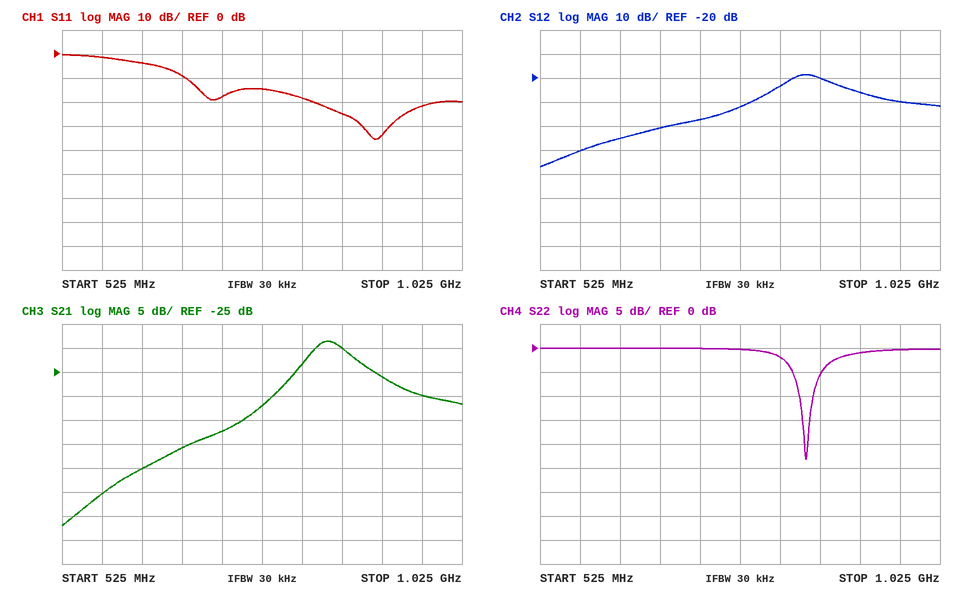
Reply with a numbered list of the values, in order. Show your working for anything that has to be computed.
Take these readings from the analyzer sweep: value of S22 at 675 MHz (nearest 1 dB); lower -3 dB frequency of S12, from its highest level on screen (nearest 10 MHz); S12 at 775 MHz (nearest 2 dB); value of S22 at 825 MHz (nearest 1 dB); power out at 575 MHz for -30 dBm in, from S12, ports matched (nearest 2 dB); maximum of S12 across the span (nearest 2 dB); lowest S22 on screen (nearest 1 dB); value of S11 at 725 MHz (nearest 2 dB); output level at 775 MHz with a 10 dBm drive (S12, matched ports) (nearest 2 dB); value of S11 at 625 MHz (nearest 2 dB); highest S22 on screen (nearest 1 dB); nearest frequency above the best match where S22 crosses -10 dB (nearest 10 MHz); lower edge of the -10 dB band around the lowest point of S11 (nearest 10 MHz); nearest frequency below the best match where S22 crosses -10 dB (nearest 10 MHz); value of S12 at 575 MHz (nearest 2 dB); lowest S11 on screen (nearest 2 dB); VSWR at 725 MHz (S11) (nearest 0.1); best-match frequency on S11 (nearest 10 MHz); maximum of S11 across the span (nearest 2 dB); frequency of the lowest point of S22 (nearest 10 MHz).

1. 0 dB
2. 830 MHz
3. -32 dB
4. -2 dB
5. -30 dBm + (-50 dB) = -80 dBm
6. -18 dB
7. -23 dB
8. -18 dB
9. 10 dBm + (-32 dB) = -22 dBm
10. -4 dB
11. 0 dB
12. 870 MHz
13. 680 MHz
14. 850 MHz
15. -50 dB
16. -36 dB
17. |Γ| = 10^(-18/20) = 0.1259; VSWR = (1 + 0.1259)/(1 − 0.1259) ≈ 1.3
18. 920 MHz
19. 0 dB
20. 860 MHz
